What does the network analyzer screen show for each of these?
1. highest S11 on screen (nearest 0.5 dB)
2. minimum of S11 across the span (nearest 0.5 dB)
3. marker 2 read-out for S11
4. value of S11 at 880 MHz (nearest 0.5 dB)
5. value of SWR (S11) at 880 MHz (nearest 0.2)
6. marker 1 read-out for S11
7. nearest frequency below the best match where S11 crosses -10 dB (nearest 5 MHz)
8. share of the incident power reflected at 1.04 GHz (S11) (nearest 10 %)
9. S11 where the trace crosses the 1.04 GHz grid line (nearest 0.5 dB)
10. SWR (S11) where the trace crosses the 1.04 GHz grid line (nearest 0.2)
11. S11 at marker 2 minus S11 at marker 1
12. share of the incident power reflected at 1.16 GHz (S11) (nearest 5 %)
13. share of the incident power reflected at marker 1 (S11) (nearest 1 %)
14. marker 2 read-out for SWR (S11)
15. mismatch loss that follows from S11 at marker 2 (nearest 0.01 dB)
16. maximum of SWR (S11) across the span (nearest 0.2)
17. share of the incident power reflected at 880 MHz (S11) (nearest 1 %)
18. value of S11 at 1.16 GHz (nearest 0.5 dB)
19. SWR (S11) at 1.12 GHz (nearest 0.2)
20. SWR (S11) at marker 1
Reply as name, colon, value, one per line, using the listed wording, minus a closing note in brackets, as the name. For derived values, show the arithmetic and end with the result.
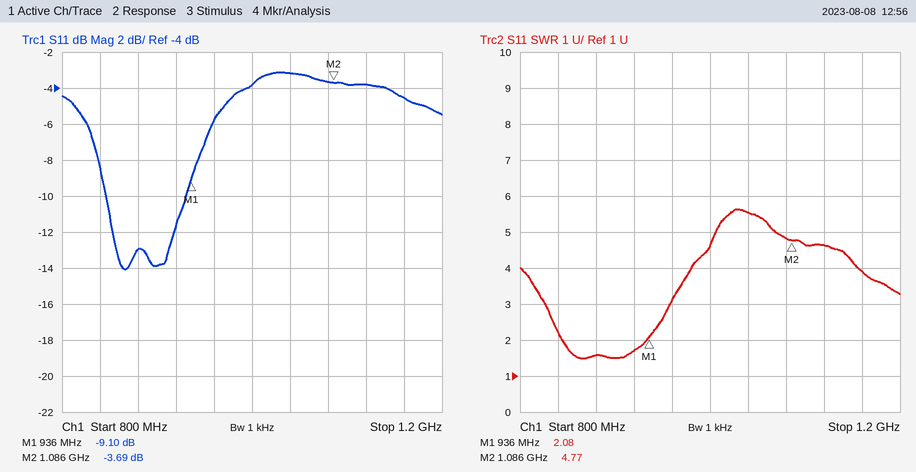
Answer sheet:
highest S11 on screen: -3.0 dB
minimum of S11 across the span: -14.0 dB
marker 2 read-out for S11: -3.69 dB
value of S11 at 880 MHz: -13.0 dB
value of SWR (S11) at 880 MHz: 1.6
marker 1 read-out for S11: -9.10 dB
nearest frequency below the best match where S11 crosses -10 dB: 845 MHz
share of the incident power reflected at 1.04 GHz (S11): 10^(-3/10) ≈ 50 %
S11 where the trace crosses the 1.04 GHz grid line: -3.0 dB
SWR (S11) where the trace crosses the 1.04 GHz grid line: 5.6
S11 at marker 2 minus S11 at marker 1: -3.69 − (-9.1) = 5.41 dB
share of the incident power reflected at 1.16 GHz (S11): 10^(-4.5/10) ≈ 35 %
share of the incident power reflected at marker 1 (S11): 10^(-9.1/10) ≈ 12 %
marker 2 read-out for SWR: 4.77
mismatch loss that follows from S11 at marker 2: −10 log10(1 − 10^(-3.69/10)) ≈ 2.42 dB
maximum of SWR (S11) across the span: 5.6
share of the incident power reflected at 880 MHz (S11): 10^(-13/10) ≈ 5 %
value of S11 at 1.16 GHz: -4.5 dB
SWR (S11) at 1.12 GHz: 4.6
SWR (S11) at marker 1: 2.08
